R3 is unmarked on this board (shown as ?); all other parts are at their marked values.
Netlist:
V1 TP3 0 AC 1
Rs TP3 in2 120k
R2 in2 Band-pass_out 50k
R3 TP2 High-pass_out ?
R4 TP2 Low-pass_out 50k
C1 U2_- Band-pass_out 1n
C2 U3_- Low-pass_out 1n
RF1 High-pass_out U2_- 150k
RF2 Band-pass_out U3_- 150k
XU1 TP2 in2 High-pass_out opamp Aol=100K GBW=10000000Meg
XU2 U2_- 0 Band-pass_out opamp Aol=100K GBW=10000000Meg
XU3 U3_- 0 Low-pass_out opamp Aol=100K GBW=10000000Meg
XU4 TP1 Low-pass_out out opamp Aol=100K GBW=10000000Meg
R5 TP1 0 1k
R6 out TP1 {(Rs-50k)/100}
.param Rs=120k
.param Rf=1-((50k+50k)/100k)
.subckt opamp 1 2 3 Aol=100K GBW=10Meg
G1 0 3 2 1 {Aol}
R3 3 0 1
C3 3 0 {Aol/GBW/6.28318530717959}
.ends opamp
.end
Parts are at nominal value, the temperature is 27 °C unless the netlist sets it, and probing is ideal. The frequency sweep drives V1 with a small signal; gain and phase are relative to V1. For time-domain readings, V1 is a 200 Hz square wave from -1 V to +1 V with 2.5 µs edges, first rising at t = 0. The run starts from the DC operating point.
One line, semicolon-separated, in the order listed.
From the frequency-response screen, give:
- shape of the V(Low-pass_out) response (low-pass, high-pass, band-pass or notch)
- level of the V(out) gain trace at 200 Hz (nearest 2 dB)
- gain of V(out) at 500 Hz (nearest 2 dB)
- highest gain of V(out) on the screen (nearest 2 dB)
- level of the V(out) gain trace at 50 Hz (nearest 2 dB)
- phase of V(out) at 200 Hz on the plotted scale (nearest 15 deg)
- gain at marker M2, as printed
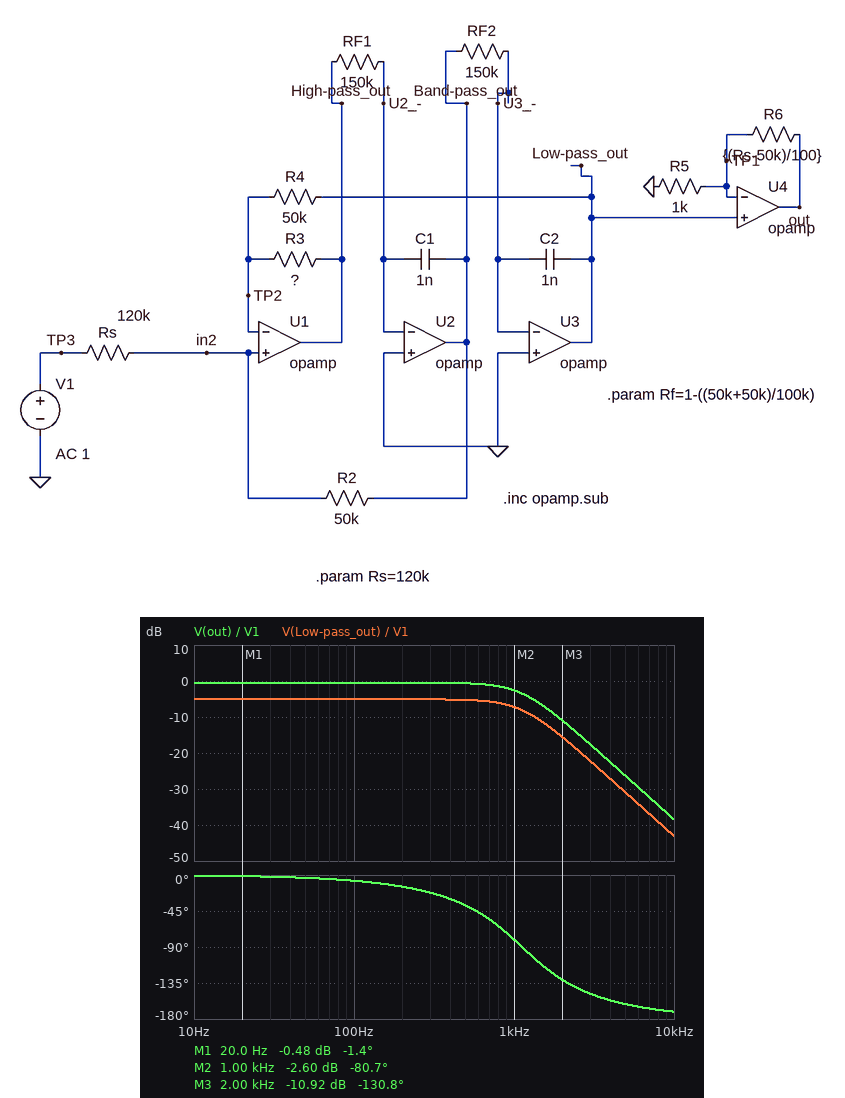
low-pass; 0 dB; 0 dB; 0 dB; 0 dB; -15 deg; -2.60 dB
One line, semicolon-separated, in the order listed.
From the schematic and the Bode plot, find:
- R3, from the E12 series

56 kΩ
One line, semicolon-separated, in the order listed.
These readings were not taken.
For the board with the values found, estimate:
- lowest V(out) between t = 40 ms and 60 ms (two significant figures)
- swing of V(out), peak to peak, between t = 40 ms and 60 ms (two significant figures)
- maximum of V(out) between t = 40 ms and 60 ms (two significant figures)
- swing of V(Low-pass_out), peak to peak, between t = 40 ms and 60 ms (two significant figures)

-1.0 V; 2.1 V; 1.0 V; 1.2 V
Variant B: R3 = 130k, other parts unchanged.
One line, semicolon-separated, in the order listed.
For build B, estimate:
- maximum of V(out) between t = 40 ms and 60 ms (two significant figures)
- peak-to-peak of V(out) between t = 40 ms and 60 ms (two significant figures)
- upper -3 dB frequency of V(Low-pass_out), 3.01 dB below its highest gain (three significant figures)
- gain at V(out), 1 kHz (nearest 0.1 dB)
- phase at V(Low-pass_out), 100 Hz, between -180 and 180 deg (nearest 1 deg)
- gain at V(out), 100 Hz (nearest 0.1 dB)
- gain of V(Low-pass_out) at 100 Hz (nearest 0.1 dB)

720 mV; 1.4 V; 1.52 kHz; -4.3 dB; -5 deg; -3.2 dB; -7.8 dB
